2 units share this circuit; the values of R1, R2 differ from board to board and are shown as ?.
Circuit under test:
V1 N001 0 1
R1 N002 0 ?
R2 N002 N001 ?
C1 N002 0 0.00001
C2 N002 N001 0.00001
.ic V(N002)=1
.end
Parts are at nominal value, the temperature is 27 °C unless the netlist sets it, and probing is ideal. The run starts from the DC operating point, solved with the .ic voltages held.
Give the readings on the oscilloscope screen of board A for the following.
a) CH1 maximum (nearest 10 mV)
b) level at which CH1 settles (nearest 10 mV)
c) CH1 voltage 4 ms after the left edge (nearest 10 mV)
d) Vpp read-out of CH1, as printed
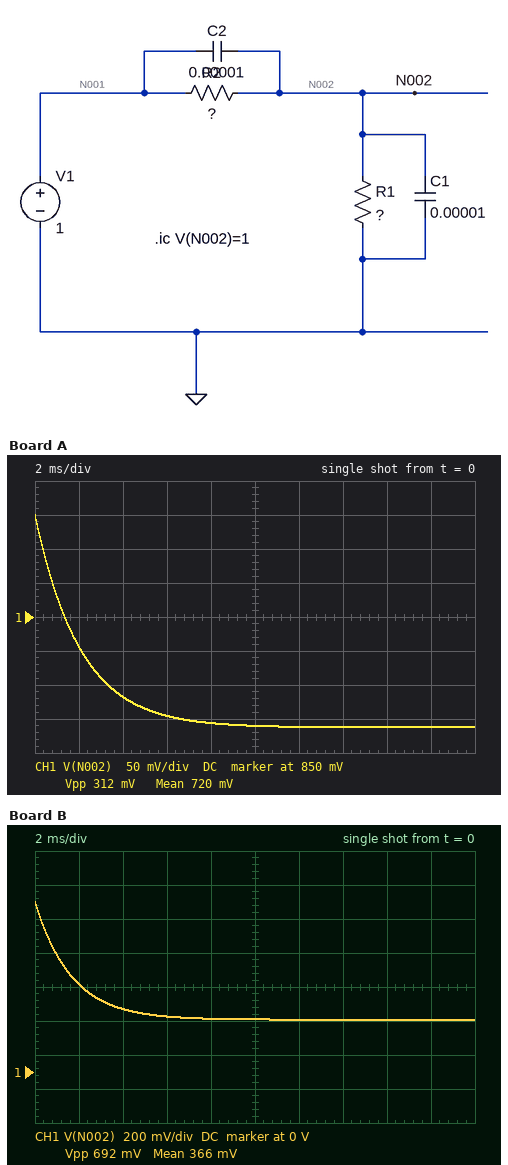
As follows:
1.00 V
690 mV
730 mV
312 mV
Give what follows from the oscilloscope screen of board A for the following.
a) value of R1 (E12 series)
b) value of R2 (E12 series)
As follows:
330 Ω
150 Ω
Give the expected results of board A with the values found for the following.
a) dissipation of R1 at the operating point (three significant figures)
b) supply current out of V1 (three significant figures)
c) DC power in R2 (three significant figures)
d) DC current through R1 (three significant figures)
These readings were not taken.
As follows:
1.43 mW
2.08 mA
651 µW
2.08 mA
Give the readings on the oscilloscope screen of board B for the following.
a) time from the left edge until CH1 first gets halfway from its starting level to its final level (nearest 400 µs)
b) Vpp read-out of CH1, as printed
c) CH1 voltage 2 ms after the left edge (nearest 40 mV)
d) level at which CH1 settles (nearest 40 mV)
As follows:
1.2 ms
692 mV
520 mV
320 mV
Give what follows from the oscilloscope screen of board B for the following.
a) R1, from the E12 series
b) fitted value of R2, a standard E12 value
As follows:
120 Ω
270 Ω
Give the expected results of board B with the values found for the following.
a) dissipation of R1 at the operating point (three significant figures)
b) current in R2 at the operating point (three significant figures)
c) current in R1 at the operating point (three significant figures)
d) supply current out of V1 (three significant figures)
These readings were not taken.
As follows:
789 µW
2.56 mA
2.56 mA
2.56 mA
